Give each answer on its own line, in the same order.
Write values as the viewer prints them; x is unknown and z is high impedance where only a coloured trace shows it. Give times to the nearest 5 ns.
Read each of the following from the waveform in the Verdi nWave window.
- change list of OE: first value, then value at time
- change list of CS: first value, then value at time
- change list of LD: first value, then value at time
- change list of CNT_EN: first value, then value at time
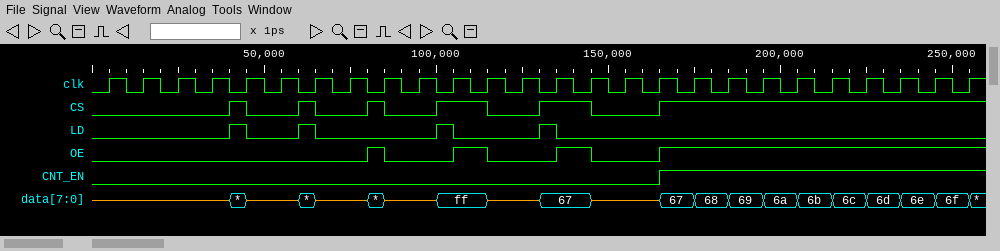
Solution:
0, 1 at 80 ns, 0 at 85 ns, 1 at 105 ns, 0 at 115 ns, 1 at 135 ns, 0 at 145 ns, 1 at 165 ns
0, 1 at 40 ns, 0 at 45 ns, 1 at 60 ns, 0 at 65 ns, 1 at 80 ns, 0 at 85 ns, 1 at 100 ns, 0 at 115 ns, 1 at 130 ns, 0 at 145 ns, 1 at 165 ns
0, 1 at 40 ns, 0 at 45 ns, 1 at 60 ns, 0 at 65 ns, 1 at 100 ns, 0 at 105 ns, 1 at 130 ns, 0 at 135 ns
0, 1 at 165 ns
